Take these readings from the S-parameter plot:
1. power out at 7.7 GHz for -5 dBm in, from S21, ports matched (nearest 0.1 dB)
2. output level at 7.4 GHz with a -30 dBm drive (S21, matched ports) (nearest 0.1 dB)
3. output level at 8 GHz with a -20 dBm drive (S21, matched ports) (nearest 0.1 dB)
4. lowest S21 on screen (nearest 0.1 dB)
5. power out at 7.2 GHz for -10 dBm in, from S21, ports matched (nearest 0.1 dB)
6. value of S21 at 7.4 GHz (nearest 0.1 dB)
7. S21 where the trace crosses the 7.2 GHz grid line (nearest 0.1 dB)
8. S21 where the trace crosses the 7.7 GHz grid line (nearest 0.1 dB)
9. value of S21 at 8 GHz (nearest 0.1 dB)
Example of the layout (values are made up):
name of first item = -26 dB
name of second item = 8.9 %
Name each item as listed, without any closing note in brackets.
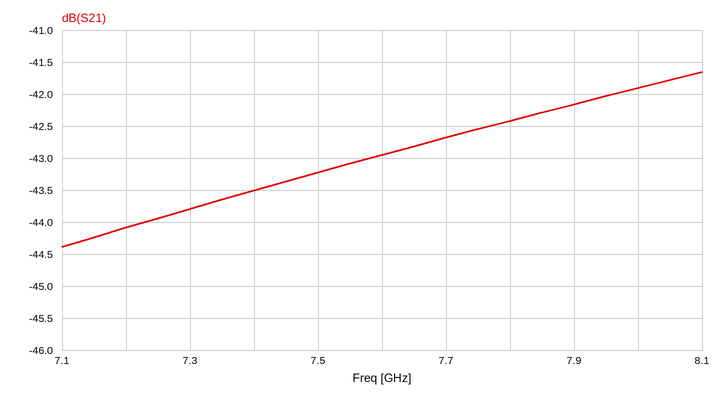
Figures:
power out at 7.7 GHz for -5 dBm in, from S21, ports matched = -47.7 dBm
output level at 7.4 GHz with a -30 dBm drive (S21, matched ports) = -73.5 dBm
output level at 8 GHz with a -20 dBm drive (S21, matched ports) = -61.9 dBm
lowest S21 on screen = -44.4 dB
power out at 7.2 GHz for -10 dBm in, from S21, ports matched = -54.1 dBm
value of S21 at 7.4 GHz = -43.5 dB
S21 where the trace crosses the 7.2 GHz grid line = -44.1 dB
S21 where the trace crosses the 7.7 GHz grid line = -42.7 dB
value of S21 at 8 GHz = -41.9 dB
